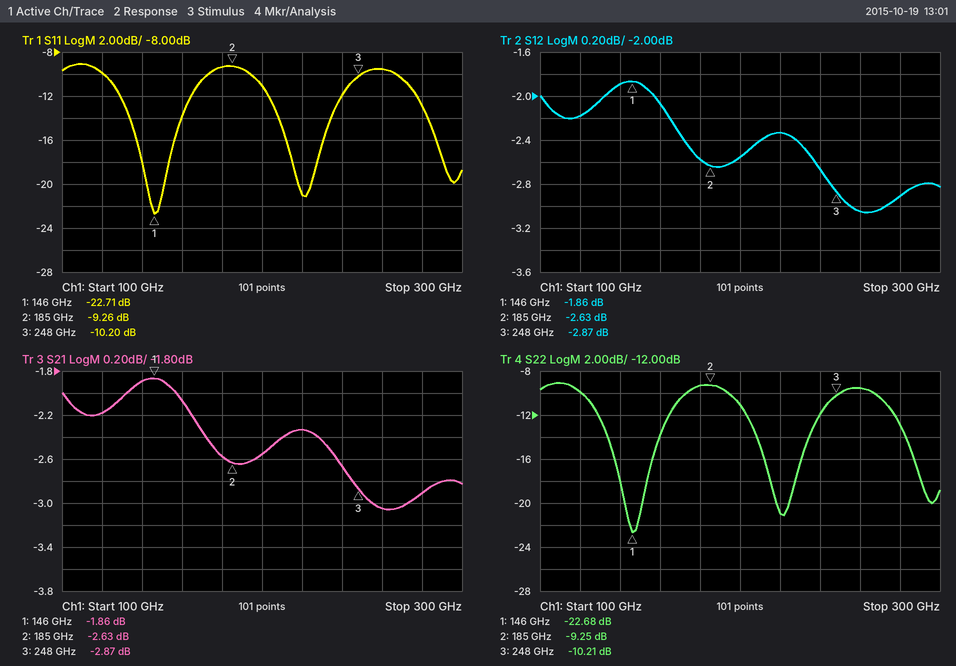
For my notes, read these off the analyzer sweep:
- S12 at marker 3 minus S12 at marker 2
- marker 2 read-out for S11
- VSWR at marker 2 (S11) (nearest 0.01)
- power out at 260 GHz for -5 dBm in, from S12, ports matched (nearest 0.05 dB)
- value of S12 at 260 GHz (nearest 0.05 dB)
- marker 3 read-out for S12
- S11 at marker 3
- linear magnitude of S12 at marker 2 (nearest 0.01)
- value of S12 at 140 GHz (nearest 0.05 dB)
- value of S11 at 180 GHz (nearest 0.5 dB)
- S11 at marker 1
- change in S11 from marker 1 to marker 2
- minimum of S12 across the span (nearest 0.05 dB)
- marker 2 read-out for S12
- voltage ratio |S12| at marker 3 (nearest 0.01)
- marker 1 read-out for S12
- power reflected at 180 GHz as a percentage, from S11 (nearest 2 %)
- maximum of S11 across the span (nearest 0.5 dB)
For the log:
-0.24 dB
-9.26 dB
2.05
-8.05 dBm
-3.05 dB
-2.87 dB
-10.20 dB
0.74
-1.90 dB
-9.5 dB
-22.71 dB
13.45 dB
-3.05 dB
-2.63 dB
0.72
-1.86 dB
12 %
-9.0 dB
